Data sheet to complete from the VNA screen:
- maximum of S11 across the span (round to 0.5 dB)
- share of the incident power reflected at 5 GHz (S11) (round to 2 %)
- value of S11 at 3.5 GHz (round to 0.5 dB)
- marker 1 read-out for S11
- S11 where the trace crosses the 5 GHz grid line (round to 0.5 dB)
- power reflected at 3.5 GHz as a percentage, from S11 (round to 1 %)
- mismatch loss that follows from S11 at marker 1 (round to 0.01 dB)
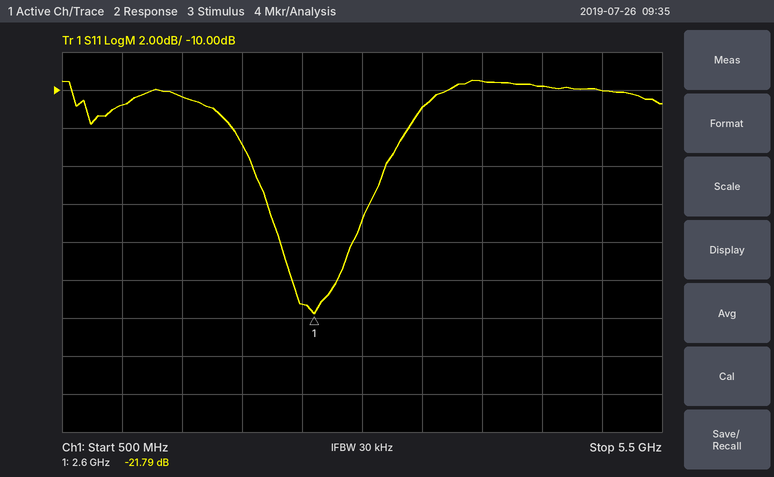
-9.5 dB
10 %
-11.0 dB
-21.79 dB
-10.0 dB
8 %
0.03 dB
